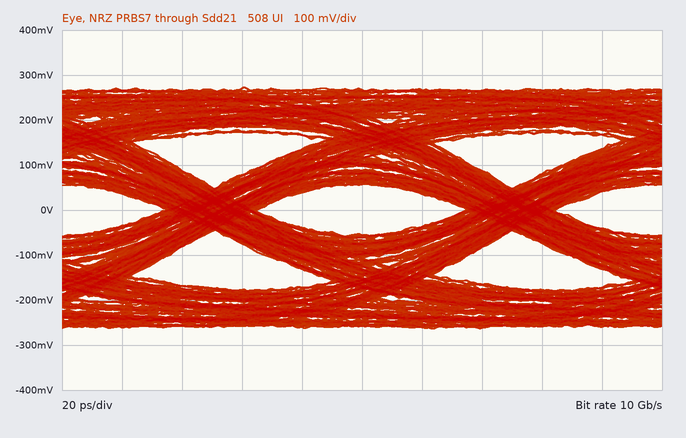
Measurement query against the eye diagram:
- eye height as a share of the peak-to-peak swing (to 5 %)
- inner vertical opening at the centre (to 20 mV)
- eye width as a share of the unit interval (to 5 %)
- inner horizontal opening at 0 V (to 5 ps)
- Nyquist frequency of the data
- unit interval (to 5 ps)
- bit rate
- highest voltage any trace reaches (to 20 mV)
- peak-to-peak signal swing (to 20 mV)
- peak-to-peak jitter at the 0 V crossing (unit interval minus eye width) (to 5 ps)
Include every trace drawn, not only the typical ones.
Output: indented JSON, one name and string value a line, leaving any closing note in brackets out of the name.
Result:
{
  "eye height as a share of the peak-to-peak swing": "20 %",
  "inner vertical opening at the centre": "120 mV",
  "eye width as a share of the unit interval": "70 %",
  "inner horizontal opening at 0 V": "70 ps",
  "Nyquist frequency of the data": "5 GHz",
  "unit interval": "100 ps",
  "bit rate": "10 Gb/s",
  "highest voltage any trace reaches": "280 mV",
  "peak-to-peak signal swing": "540 mV",
  "peak-to-peak jitter at the 0 V crossing (unit interval minus eye width)": "30 ps"
}
